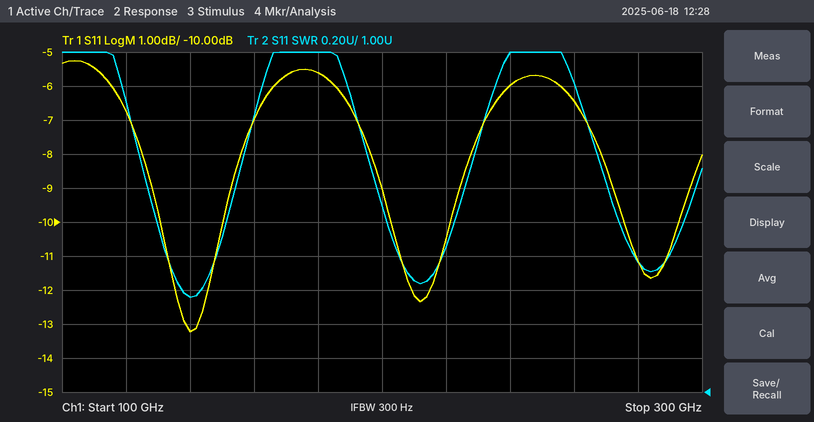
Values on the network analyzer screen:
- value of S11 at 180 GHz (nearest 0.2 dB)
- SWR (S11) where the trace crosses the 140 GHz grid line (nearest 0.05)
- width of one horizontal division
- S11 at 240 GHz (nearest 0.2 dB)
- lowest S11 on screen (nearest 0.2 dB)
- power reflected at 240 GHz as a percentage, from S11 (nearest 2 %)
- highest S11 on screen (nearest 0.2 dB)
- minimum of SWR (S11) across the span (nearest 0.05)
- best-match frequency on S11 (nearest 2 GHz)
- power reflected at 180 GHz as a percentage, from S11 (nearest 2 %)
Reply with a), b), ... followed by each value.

a) -5.6 dB
b) 1.55
c) 20 GHz
d) -6.0 dB
e) -13.2 dB
f) 26 %
g) -5.2 dB
h) 1.55
i) 140 GHz
j) 28 %
